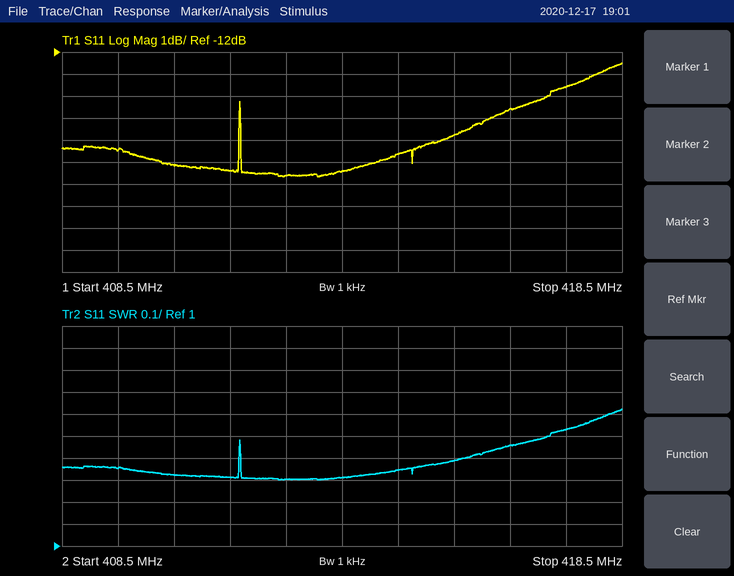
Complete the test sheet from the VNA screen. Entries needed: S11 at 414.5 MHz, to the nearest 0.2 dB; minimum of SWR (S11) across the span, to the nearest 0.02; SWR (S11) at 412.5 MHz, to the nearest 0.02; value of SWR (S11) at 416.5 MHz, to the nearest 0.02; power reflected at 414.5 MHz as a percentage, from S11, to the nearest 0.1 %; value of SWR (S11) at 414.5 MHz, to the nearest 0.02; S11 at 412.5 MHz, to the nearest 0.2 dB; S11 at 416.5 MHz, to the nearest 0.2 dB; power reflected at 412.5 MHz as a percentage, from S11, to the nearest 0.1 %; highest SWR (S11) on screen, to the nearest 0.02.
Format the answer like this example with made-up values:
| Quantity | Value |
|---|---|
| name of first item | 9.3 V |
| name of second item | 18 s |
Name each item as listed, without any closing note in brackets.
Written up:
| Quantity | Value |
|---|---|
| S11 at 414.5 MHz, to the nearest 0.2 dB | -16.6 dB |
| minimum of SWR (S11) across the span, to the nearest 0.02 | 1.30 |
| SWR (S11) at 412.5 MHz, to the nearest 0.02 | 1.30 |
| value of SWR (S11) at 416.5 MHz, to the nearest 0.02 | 1.46 |
| power reflected at 414.5 MHz as a percentage, from S11, to the nearest 0.1 % | 2.2 % |
| value of SWR (S11) at 414.5 MHz, to the nearest 0.02 | 1.34 |
| S11 at 412.5 MHz, to the nearest 0.2 dB | -17.6 dB |
| S11 at 416.5 MHz, to the nearest 0.2 dB | -14.6 dB |
| power reflected at 412.5 MHz as a percentage, from S11, to the nearest 0.1 % | 1.7 % |
| highest SWR (S11) on screen, to the nearest 0.02 | 1.62 |
